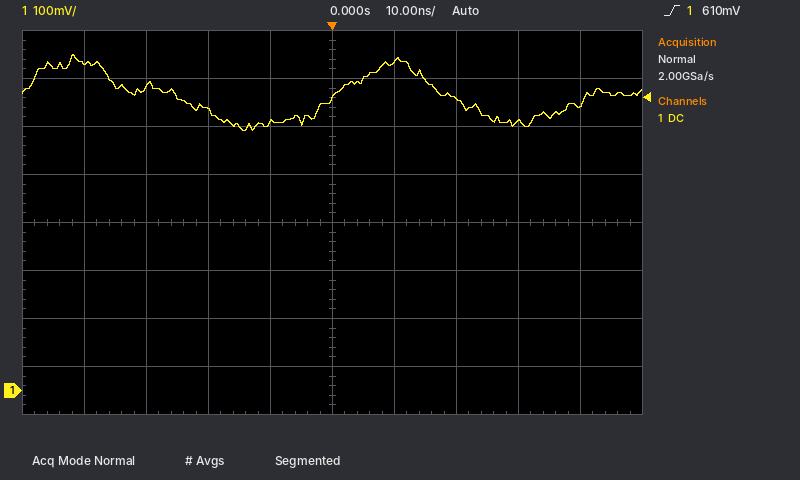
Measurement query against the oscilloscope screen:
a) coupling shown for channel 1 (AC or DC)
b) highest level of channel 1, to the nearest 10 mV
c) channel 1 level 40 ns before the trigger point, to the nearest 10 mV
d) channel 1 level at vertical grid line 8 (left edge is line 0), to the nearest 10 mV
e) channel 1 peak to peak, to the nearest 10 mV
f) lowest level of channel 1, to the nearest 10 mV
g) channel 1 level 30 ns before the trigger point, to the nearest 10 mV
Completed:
DC
700 mV
680 mV
560 mV
160 mV
540 mV
630 mV
